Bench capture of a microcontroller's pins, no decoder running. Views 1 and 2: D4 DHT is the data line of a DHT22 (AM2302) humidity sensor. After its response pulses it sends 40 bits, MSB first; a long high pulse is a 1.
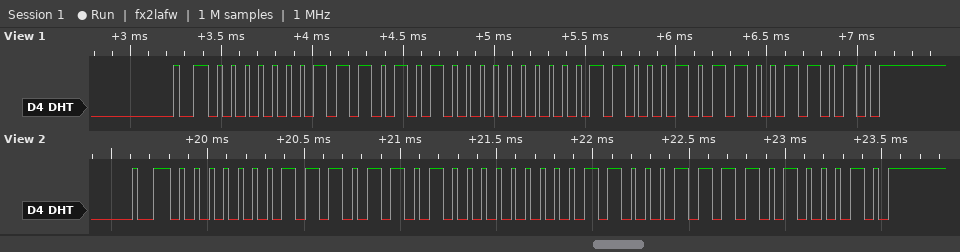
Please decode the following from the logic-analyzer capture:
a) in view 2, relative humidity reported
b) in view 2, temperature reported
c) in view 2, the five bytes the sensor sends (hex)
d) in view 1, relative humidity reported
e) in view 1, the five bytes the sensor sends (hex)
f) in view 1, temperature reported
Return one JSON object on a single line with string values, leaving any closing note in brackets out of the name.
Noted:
{"in view 2, relative humidity reported": "47.4 %", "in view 2, temperature reported": "19.9 °C", "in view 2, the five bytes the sensor sends": "01 DA 00 C7 A2", "in view 1, relative humidity reported": "46.8 %", "in view 1, the five bytes the sensor sends": "01 D4 00 C5 9A", "in view 1, temperature reported": "19.7 °C"}
